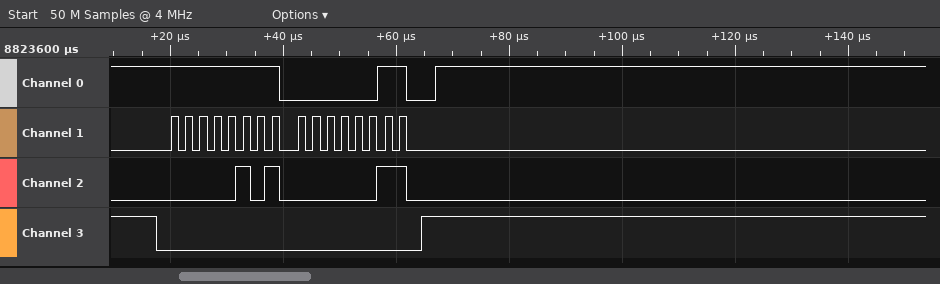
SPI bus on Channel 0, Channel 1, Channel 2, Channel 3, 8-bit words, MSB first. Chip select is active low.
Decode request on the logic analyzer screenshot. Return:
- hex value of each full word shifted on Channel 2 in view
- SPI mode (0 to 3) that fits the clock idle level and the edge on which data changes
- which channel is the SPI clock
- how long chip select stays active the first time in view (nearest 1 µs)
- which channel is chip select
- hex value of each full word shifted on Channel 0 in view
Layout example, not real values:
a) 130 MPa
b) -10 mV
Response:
a) 05, 03
b) 0
c) Channel 1
d) 47 µs
e) Channel 3
f) FF, 03
